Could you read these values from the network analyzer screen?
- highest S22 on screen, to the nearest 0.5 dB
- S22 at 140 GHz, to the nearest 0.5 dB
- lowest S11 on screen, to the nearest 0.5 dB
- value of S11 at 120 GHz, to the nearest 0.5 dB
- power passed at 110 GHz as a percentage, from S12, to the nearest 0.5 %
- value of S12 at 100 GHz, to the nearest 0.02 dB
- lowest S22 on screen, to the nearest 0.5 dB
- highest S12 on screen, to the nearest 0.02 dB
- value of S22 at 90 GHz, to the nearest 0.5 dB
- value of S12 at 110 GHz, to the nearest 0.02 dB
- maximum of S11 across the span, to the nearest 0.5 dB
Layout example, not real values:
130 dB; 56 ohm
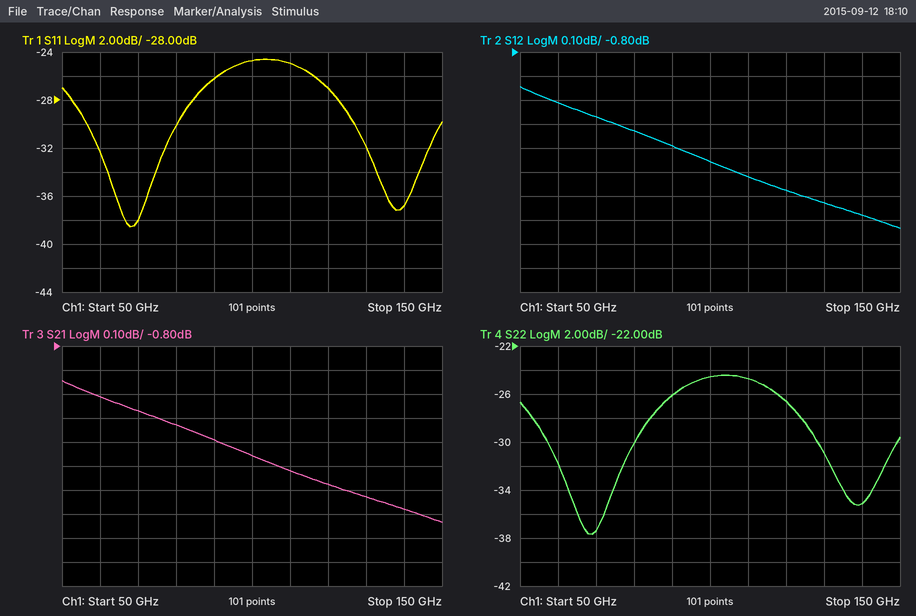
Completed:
-24.5 dB; -35.0 dB; -38.5 dB; -27.0 dB; 74.0 %; -1.26 dB; -37.5 dB; -0.94 dB; -26.0 dB; -1.32 dB; -24.5 dB
